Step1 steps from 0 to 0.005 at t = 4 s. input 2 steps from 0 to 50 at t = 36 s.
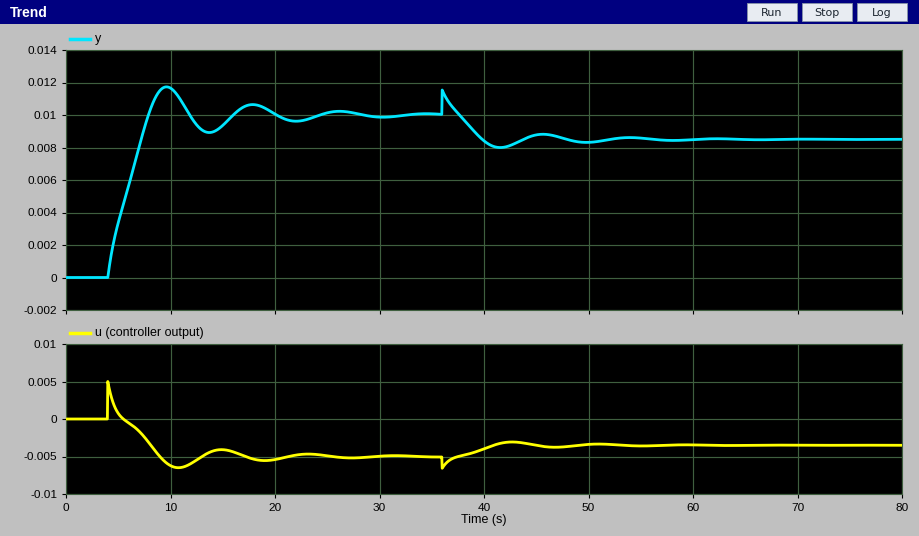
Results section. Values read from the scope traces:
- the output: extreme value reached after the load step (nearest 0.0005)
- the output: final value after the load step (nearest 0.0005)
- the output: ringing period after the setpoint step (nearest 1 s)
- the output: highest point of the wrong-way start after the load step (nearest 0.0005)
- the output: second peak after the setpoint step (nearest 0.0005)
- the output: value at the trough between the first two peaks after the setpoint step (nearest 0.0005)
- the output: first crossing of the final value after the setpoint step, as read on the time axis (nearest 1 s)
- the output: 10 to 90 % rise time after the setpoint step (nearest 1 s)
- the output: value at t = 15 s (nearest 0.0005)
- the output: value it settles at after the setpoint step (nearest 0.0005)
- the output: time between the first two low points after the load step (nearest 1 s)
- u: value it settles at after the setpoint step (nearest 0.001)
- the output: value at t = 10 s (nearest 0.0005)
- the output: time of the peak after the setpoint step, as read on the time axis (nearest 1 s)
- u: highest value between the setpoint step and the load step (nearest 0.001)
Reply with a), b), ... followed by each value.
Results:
a) 0.0080
b) 0.0085
c) 8 s
d) 0.0115
e) 0.0105
f) 0.0090
g) 8 s
h) 3 s
i) 0.0095
j) 0.0100
k) 8 s
l) -0.005
m) 0.0115
n) 10 s
o) 0.005
